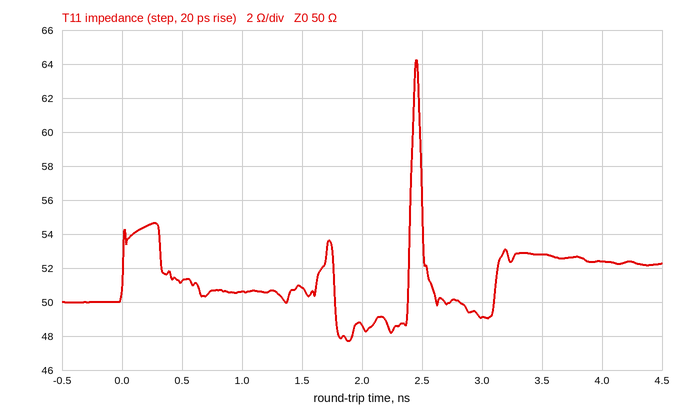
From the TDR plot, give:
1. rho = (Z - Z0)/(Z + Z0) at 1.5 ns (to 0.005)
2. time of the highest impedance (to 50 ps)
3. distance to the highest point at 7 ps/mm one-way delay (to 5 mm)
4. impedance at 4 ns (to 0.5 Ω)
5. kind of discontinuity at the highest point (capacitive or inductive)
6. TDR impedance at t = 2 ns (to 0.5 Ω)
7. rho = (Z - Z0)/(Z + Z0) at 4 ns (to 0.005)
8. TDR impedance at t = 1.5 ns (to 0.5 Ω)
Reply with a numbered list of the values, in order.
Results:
1. +0.010
2. 2.45 ns
3. 175 mm
4. 52.5 Ω
5. inductive
6. 48.5 Ω
7. +0.025
8. 51.0 Ω
